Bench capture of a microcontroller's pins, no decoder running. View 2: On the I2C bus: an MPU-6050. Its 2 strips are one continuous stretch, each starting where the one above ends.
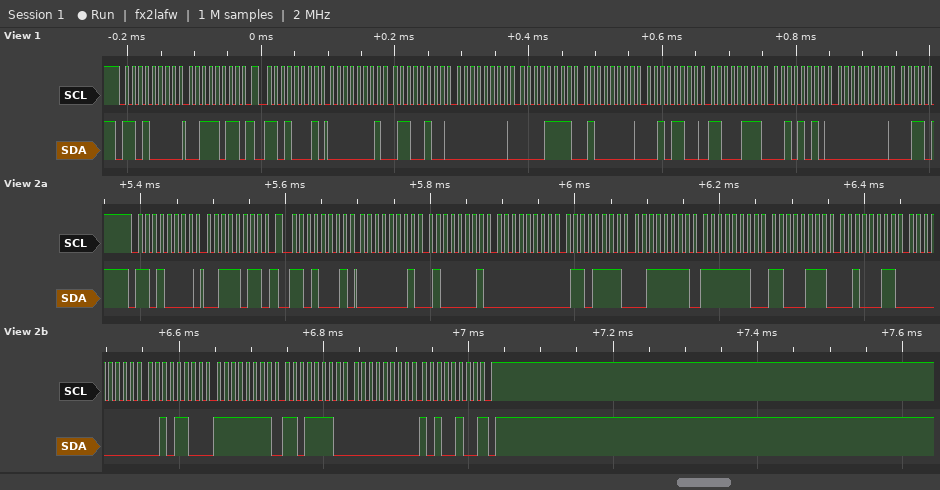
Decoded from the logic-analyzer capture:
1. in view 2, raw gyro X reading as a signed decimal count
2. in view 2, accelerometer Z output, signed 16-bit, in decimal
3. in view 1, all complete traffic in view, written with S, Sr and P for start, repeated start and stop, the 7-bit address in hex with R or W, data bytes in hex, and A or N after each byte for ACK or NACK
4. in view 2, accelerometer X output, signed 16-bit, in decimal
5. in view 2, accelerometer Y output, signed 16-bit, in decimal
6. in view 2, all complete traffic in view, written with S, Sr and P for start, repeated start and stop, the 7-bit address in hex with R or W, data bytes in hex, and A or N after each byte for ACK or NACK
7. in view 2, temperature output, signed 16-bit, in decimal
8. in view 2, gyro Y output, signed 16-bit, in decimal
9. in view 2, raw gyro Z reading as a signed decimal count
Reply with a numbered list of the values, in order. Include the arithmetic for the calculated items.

1. 0x002C = 44
2. 0x3FFE = 16382
3. S 68W A 3B A Sr 68R A 01 A 64 A 00 A 0F A 40 A 2C A C7 A 2A A 00 A
4. 0x0141 = 321
5. 0x006F = 111
6. S 68W A 3B A Sr 68R A 01 A 41 A 00 A 6F A 3F A FE A C7 A 23 A 00 A 2C A FF A DE A 00 A A4 N P
7. 0xC723 = -14557
8. 0xFFDE = -34
9. 0x00A4 = 164
